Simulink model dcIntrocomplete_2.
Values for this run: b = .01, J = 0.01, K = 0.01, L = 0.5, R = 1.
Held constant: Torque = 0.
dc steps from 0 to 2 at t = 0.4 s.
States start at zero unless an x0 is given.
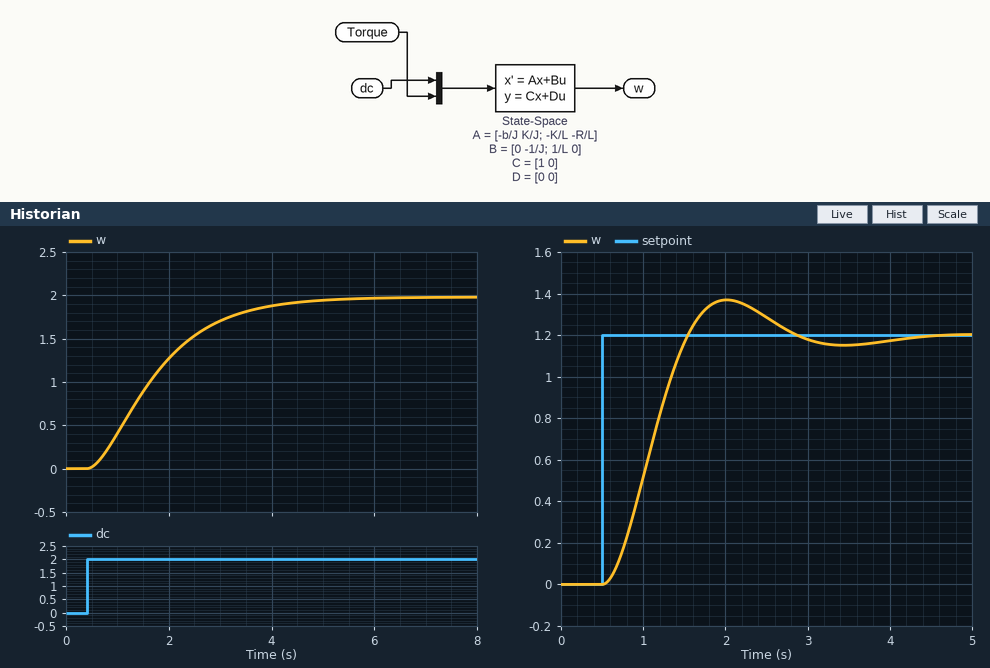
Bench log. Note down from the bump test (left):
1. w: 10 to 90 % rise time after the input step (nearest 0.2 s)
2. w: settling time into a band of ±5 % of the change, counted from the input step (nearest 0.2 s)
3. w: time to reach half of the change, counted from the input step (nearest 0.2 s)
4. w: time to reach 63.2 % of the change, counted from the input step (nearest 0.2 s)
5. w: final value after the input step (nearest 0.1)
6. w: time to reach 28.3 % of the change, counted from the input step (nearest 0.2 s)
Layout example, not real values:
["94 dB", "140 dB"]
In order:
["2.6 s", "3.6 s", "1.2 s", "1.6 s", "2.0", "0.8 s"]
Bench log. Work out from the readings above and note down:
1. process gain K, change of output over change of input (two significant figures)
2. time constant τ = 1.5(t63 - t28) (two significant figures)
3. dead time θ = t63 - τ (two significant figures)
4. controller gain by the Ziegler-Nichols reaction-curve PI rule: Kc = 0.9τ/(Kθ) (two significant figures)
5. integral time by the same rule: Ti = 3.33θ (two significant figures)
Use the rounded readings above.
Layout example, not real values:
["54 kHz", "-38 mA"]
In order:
["1.0", "1.2 s", "0.40 s", "2.7", "1.3 s"]
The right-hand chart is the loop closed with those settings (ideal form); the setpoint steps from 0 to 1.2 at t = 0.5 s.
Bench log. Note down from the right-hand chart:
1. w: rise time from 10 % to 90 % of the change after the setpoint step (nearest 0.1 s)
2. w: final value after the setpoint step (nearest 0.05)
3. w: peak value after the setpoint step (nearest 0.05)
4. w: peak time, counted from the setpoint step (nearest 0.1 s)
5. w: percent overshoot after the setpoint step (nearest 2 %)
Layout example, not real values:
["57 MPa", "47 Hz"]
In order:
["0.7 s", "1.20", "1.35", "1.5 s", "14 %"]
